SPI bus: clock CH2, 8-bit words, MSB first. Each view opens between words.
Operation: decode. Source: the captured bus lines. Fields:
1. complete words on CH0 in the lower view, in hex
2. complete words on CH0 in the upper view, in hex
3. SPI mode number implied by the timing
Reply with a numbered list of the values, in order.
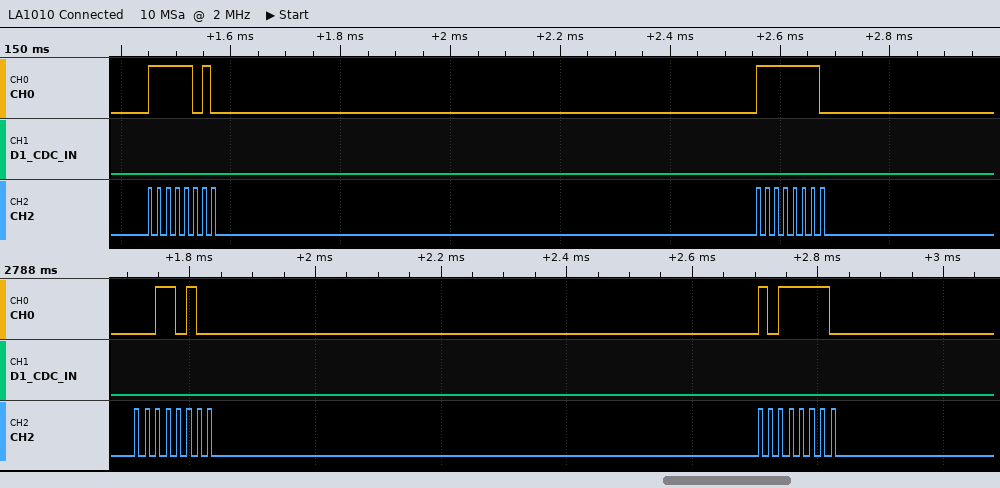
1. 34, BE
2. FA, FE
3. 1
